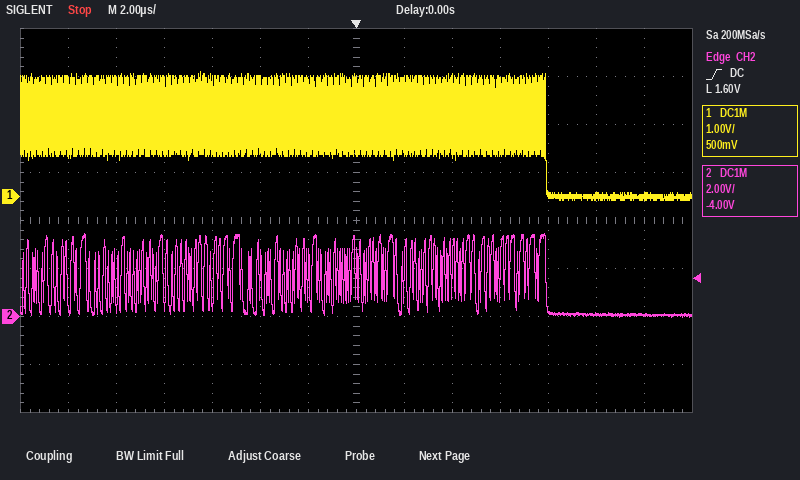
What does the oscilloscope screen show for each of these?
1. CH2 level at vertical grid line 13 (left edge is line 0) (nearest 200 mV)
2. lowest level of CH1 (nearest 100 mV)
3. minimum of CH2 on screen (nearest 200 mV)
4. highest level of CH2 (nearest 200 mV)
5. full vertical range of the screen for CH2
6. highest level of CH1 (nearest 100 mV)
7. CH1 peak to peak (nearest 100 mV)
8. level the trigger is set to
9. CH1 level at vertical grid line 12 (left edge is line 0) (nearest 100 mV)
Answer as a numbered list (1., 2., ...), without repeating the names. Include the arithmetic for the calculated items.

1. 0.0 V
2. -100 mV
3. 0.0 V
4. 3.4 V
5. 16 V
6. 2.6 V
7. 2.6 V − (-100 mV) = 2.7 V
8. 1.60 V
9. 0.0 V
